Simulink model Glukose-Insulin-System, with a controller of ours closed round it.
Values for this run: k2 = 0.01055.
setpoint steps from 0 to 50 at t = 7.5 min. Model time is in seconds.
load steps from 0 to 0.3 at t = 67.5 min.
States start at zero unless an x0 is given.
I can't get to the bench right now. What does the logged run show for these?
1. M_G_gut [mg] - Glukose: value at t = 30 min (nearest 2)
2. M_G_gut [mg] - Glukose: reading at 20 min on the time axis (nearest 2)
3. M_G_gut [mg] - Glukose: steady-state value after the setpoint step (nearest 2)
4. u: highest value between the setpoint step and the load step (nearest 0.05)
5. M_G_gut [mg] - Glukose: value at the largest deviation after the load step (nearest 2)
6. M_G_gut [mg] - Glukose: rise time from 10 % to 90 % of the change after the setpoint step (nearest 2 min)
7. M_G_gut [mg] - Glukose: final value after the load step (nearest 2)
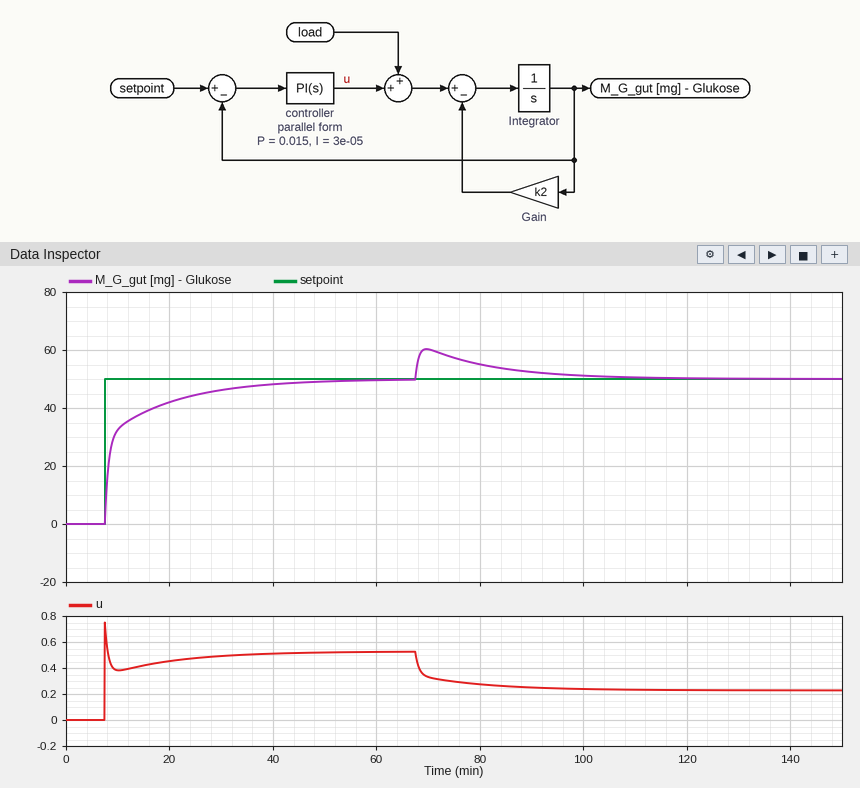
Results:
46
42
50
0.75
60
18 min
50
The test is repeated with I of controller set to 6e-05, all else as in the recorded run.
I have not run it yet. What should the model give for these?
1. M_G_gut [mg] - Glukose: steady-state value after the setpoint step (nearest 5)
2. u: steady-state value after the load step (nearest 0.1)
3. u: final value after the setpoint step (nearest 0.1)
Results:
50
0.2
0.5
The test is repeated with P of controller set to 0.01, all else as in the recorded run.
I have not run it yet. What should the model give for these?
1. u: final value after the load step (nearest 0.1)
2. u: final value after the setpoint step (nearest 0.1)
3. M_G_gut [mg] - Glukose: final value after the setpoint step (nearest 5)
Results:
0.2
0.5
50
